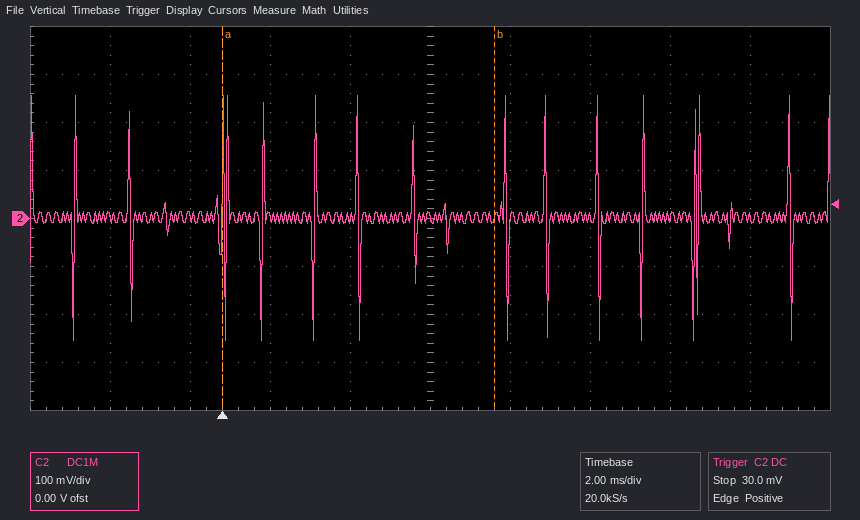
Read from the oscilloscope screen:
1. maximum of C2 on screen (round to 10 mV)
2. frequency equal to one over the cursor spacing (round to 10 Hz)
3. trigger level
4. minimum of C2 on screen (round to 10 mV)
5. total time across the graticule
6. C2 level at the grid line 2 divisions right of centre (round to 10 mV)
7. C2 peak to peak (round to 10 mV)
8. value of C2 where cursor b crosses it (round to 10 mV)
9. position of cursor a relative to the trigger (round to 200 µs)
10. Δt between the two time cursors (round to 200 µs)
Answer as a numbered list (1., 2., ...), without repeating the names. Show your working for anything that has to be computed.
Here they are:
1. 260 mV
2. 1 / 6.8 ms ≈ 150 Hz
3. 30.0 mV
4. -250 mV
5. 20 ms
6. 0 mV
7. 260 mV − (-250 mV) = 510 mV
8. 0 mV
9. 0.0 ms
10. 6.8 ms
